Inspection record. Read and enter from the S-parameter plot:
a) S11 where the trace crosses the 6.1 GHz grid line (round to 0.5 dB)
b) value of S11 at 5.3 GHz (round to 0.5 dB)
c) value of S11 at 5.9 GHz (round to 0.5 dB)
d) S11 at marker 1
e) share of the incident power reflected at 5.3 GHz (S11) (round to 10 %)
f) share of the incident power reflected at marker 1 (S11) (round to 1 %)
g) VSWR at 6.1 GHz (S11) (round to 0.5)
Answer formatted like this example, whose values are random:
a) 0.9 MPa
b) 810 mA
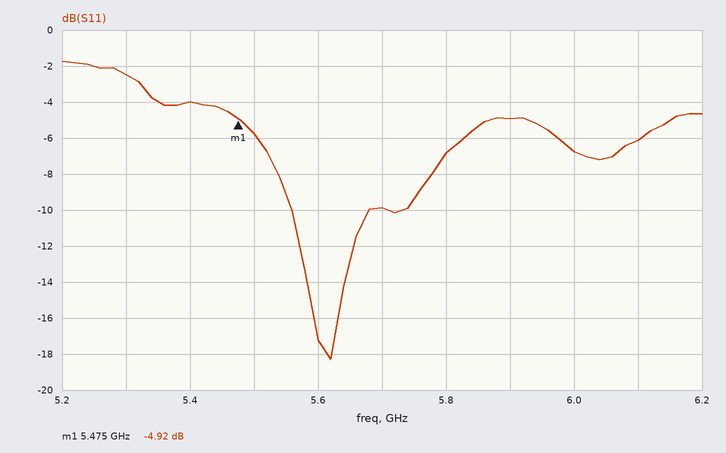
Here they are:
a) -6.0 dB
b) -2.5 dB
c) -5.0 dB
d) -4.92 dB
e) 60 %
f) 32 %
g) 3.0
